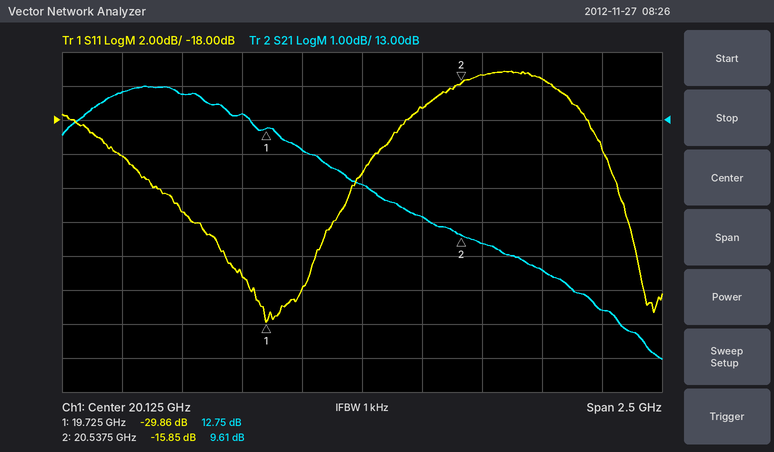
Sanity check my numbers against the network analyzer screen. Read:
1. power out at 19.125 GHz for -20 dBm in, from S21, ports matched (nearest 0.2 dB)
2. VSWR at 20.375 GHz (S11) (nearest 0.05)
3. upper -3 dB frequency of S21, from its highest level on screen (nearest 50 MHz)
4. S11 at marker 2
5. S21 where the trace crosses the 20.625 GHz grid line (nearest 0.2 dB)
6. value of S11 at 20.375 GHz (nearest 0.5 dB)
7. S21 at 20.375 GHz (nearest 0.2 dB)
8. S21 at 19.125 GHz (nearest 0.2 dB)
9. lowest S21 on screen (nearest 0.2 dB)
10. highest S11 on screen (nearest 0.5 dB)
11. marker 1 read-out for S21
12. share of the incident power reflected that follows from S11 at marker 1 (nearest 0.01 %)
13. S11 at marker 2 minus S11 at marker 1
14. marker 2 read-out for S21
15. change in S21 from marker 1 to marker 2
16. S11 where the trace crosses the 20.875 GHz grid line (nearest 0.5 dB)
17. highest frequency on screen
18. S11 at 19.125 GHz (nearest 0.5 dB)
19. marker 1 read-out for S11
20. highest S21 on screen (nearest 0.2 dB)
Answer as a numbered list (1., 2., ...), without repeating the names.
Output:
1. -6.2 dBm
2. 1.30
3. 20.15 GHz
4. -15.85 dB
5. 9.4 dB
6. -17.5 dB
7. 10.2 dB
8. 13.8 dB
9. 6.0 dB
10. -15.0 dB
11. 12.75 dB
12. 0.10 %
13. 14.01 dB
14. 9.61 dB
15. -3.14 dB
16. -15.5 dB
17. 21.375 GHz
18. -20.0 dB
19. -29.86 dB
20. 14.0 dB
